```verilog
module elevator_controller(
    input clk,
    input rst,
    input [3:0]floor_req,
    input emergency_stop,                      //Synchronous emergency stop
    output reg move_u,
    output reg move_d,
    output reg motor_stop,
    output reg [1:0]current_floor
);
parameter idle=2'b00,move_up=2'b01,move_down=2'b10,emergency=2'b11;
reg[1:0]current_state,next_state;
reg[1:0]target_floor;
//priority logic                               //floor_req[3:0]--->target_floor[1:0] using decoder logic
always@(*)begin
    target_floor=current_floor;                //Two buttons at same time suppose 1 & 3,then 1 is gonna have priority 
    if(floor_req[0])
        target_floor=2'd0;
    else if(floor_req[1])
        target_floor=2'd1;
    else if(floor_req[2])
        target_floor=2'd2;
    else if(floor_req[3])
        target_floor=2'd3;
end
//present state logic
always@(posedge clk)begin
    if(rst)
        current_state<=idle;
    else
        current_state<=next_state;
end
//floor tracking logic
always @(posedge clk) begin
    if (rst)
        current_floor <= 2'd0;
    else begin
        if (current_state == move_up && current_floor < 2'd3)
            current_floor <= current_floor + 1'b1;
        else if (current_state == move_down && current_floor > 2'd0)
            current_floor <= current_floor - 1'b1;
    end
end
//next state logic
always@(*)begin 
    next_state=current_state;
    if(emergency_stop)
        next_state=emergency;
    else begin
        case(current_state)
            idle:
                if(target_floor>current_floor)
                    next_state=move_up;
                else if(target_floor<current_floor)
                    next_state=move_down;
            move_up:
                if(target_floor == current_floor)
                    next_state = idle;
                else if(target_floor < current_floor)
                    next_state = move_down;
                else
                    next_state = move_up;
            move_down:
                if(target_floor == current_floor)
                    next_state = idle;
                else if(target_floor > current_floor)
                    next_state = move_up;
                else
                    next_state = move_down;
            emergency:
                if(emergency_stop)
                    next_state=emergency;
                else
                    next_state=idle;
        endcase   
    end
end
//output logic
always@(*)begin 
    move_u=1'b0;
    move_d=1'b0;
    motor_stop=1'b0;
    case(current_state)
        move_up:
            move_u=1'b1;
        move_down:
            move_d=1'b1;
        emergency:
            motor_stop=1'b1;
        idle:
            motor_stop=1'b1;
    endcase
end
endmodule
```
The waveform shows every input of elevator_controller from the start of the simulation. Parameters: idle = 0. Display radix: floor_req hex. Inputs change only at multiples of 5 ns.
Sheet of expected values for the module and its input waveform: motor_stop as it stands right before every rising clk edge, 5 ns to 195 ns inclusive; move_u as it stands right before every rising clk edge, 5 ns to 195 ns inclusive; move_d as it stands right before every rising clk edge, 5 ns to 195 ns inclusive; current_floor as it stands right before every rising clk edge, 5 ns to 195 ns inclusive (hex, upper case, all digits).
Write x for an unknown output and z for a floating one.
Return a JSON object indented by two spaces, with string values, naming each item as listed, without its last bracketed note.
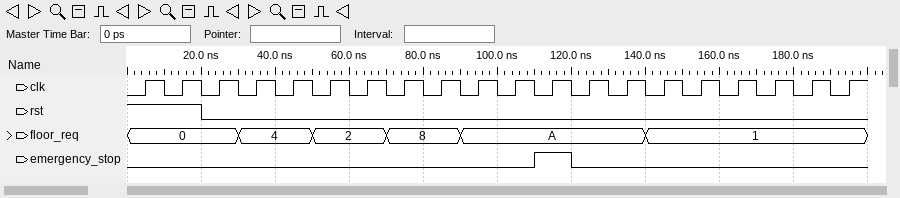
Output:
{
  "motor_stop as it stands right before every rising clk edge, 5 ns to 195 ns inclusive": "x 1 1 1 0 0 1 0 0 0 0 0 1 1 1 0 0 1 1 1",
  "move_u as it stands right before every rising clk edge, 5 ns to 195 ns inclusive": "x 0 0 0 1 1 0 0 1 1 0 0 0 0 0 0 0 0 0 0",
  "move_d as it stands right before every rising clk edge, 5 ns to 195 ns inclusive": "x 0 0 0 0 0 0 1 0 0 1 1 0 0 0 1 1 0 0 0",
  "current_floor as it stands right before every rising clk edge, 5 ns to 195 ns inclusive": "x, 0, 0, 0, 0, 1, 2, 2, 1, 2, 3, 2, 1, 1, 1, 1, 0, 0, 0, 0"
}
